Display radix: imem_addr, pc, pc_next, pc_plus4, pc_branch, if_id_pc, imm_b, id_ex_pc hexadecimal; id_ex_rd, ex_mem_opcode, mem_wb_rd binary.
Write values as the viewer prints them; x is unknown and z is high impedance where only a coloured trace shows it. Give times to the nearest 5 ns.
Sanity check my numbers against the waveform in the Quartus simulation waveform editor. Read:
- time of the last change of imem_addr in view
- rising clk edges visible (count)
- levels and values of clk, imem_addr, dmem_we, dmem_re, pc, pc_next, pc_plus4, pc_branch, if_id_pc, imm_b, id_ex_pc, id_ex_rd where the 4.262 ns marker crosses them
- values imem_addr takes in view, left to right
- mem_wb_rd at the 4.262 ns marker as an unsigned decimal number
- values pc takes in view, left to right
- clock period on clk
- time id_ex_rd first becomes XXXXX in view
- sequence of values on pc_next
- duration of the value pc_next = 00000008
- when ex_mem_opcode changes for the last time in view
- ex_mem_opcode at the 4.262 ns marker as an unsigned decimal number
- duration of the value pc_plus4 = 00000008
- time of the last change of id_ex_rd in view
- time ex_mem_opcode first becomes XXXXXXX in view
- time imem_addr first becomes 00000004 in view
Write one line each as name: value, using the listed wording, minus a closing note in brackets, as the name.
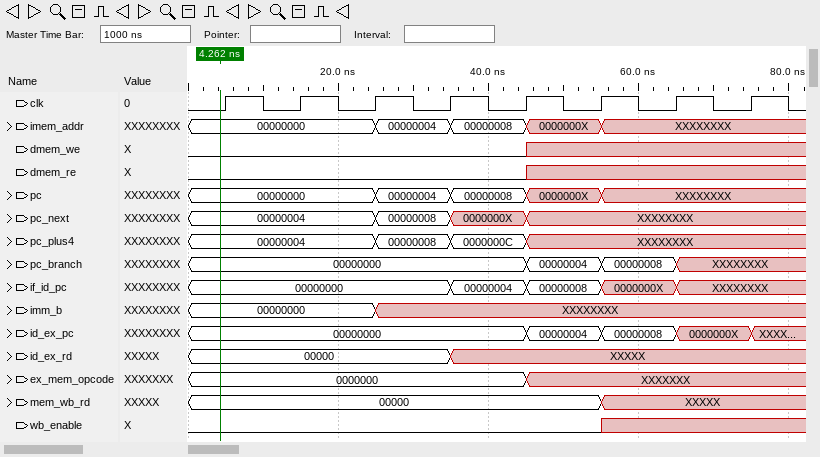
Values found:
time of the last change of imem_addr in view: 55 ns
rising clk edges visible: 8
levels and values of clk, imem_addr, dmem_we, dmem_re, pc, pc_next, pc_plus4, pc_branch, if_id_pc, imm_b, id_ex_pc, id_ex_rd where the 4.262 ns marker crosses them: clk=0, imem_addr=00000000, dmem_we=0, dmem_re=0, pc=00000000, pc_next=00000004, pc_plus4=00000004, pc_branch=00000000, if_id_pc=00000000, imm_b=00000000, id_ex_pc=00000000, id_ex_rd=00000
values imem_addr takes in view, left to right: 00000000, 00000004, 00000008, 0000000X, XXXXXXXX
mem_wb_rd at the 4.262 ns marker as an unsigned decimal number: 0
values pc takes in view, left to right: 00000000, 00000004, 00000008, 0000000X, XXXXXXXX
clock period on clk: 10 ns
time id_ex_rd first becomes XXXXX in view: 35 ns
sequence of values on pc_next: 00000004, 00000008, 0000000X, XXXXXXXX
duration of the value pc_next = 00000008: 10 ns
when ex_mem_opcode changes for the last time in view: 45 ns
ex_mem_opcode at the 4.262 ns marker as an unsigned decimal number: 0
duration of the value pc_plus4 = 00000008: 10 ns
time of the last change of id_ex_rd in view: 35 ns
time ex_mem_opcode first becomes XXXXXXX in view: 45 ns
time imem_addr first becomes 00000004 in view: 25 ns
